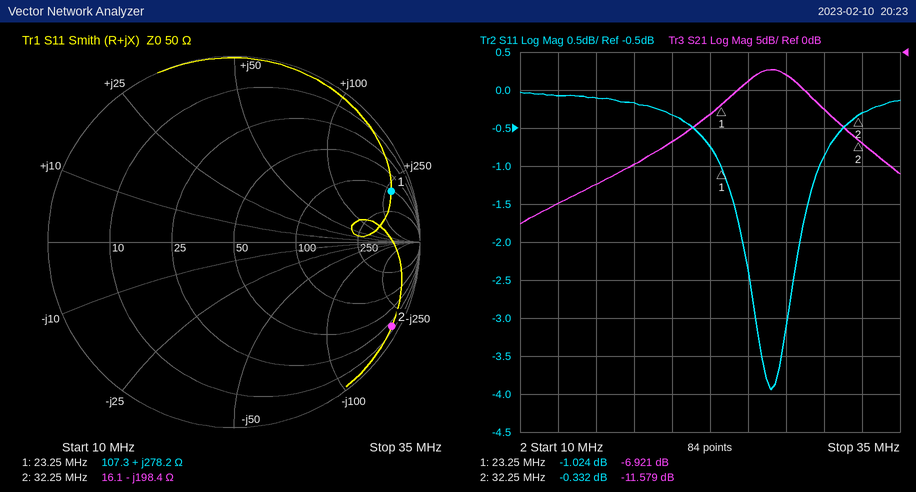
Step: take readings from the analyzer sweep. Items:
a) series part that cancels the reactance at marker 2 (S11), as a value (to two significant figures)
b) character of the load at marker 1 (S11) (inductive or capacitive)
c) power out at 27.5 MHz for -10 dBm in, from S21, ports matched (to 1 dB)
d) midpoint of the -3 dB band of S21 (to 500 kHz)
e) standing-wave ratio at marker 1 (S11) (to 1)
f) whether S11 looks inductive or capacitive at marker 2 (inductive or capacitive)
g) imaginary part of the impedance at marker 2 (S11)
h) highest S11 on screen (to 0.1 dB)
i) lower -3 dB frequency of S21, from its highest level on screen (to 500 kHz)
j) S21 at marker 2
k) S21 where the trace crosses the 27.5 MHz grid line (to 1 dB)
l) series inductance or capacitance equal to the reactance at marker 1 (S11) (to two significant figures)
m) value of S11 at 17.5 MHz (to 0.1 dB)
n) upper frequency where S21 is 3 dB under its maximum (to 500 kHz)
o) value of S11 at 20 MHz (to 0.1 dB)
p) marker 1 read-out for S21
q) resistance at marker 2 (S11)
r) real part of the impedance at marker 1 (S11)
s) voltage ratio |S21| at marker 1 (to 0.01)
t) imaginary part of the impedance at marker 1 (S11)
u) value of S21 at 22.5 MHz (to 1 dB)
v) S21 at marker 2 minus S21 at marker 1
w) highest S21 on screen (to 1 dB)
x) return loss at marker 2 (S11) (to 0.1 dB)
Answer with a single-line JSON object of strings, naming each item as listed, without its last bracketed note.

{"series part that cancels the reactance at marker 2 (S11), as a value": "980 nH", "character of the load at marker 1 (S11)": "inductive", "power out at 27.5 MHz for -10 dBm in, from S21, ports matched": "-13 dBm", "midpoint of the -3 dB band of S21": "26.5 MHz", "standing-wave ratio at marker 1 (S11)": "17", "whether S11 looks inductive or capacitive at marker 2": "capacitive", "imaginary part of the impedance at marker 2": "-198.4 Ω", "highest S11 on screen": "0.0 dB", "lower -3 dB frequency of S21, from its highest level on screen": "24.0 MHz", "S21 at marker 2": "-11.579 dB", "S21 where the trace crosses the 27.5 MHz grid line": "-3 dB", "series inductance or capacitance equal to the reactance at marker 1 (S11)": "1.9 µH", "value of S11 at 17.5 MHz": "-0.2 dB", "upper frequency where S21 is 3 dB under its maximum": "29.0 MHz", "value of S11 at 20 MHz": "-0.3 dB", "marker 1 read-out for S21": "-6.921 dB", "resistance at marker 2": "16.1 Ω", "real part of the impedance at marker 1": "107.3 Ω", "voltage ratio |S21| at marker 1": "0.45", "imaginary part of the impedance at marker 1": "+278.2 Ω", "value of S21 at 22.5 MHz": "-8 dB", "S21 at marker 2 minus S21 at marker 1": "-4.658 dB", "highest S21 on screen": "-2 dB", "return loss at marker 2 (S11)": "0.3 dB"}
